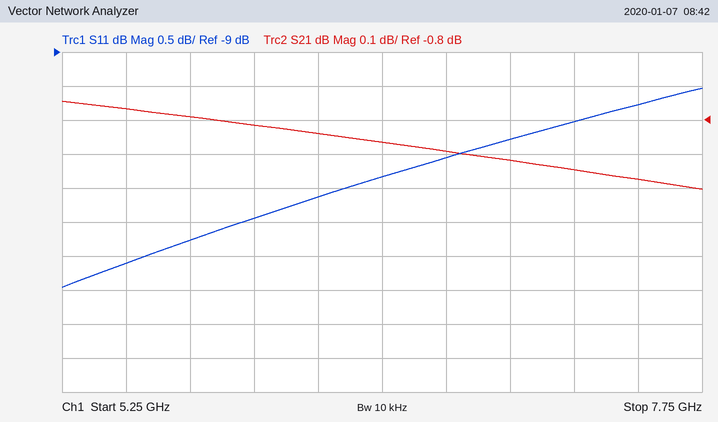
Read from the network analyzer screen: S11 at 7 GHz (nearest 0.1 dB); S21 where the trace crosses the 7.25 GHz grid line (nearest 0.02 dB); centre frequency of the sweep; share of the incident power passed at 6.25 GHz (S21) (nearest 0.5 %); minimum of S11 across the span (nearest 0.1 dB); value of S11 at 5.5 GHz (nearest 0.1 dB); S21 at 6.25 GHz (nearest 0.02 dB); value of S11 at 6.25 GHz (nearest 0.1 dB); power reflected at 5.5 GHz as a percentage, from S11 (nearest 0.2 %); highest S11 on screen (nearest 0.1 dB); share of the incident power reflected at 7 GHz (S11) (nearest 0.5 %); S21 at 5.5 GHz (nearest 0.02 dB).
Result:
-10.3 dB
-0.94 dB
6.5 GHz
82.5 %
-12.5 dB
-12.1 dB
-0.84 dB
-11.1 dB
6.2 %
-9.5 dB
9.5 %
-0.76 dB
